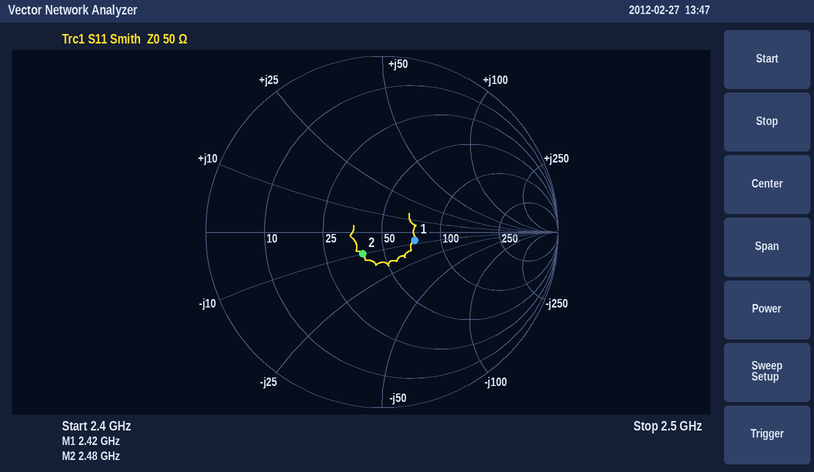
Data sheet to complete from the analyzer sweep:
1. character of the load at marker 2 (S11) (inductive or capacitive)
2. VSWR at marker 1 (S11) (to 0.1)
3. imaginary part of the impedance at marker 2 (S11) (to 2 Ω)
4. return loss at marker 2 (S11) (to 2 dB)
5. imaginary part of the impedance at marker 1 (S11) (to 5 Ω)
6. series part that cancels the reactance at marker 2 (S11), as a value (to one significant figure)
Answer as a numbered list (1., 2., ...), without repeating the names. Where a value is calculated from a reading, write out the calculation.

1. capacitive
2. 1.5
3. -10 Ω
4. 16 dB
5. -5 Ω
6. L = 10 Ω/(2π × 2.48 GHz) ≈ 642 pH, so 600 pH to one significant figure
